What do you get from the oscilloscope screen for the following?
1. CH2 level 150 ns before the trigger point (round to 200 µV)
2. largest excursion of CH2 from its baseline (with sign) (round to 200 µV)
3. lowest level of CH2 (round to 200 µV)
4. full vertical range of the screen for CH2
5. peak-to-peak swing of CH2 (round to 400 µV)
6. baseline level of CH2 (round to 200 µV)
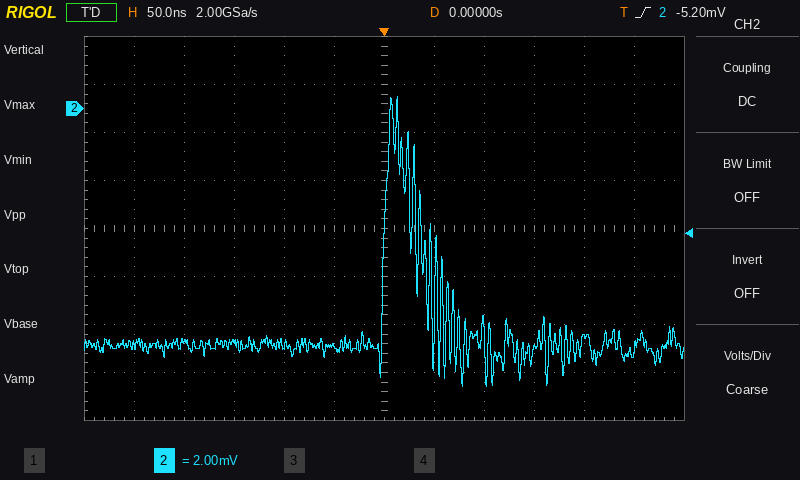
-9.8 mV
+10.4 mV
-11.6 mV
16 mV
12.0 mV
-9.8 mV
